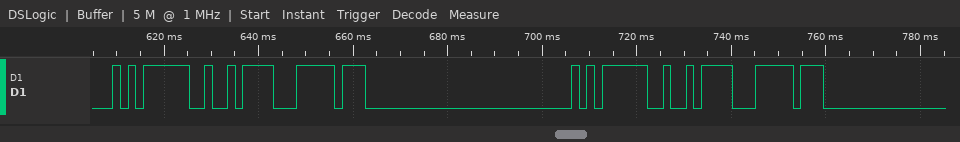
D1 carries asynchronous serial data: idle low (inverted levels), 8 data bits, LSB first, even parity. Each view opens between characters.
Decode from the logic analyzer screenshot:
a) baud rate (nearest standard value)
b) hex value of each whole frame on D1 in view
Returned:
600 baud
05, 0B, 10, 05, 0B, 10
